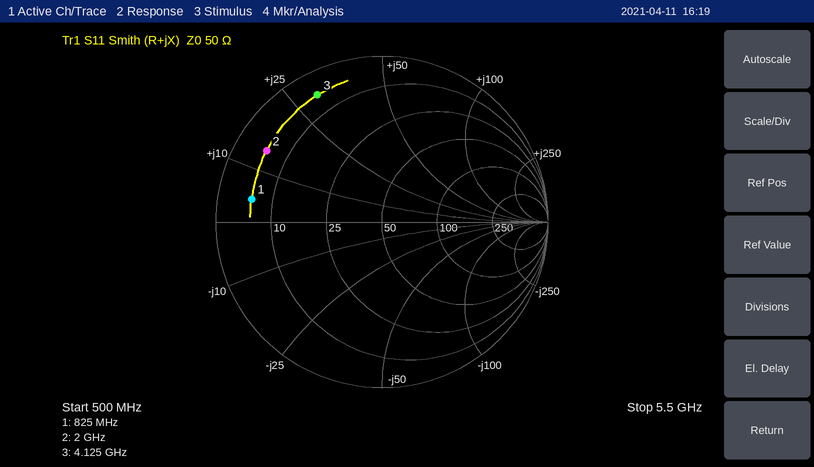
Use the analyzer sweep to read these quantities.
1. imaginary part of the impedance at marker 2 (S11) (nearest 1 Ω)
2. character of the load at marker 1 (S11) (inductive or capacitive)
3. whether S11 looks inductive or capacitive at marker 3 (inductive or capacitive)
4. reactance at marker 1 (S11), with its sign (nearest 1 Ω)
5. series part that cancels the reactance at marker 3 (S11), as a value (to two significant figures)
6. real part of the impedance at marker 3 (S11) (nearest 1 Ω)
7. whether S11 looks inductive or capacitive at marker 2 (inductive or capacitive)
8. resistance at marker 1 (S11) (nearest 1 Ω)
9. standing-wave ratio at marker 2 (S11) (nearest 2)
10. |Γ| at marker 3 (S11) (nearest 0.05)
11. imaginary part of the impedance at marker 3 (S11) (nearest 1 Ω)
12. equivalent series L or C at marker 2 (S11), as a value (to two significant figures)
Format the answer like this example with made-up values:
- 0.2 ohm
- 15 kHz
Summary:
- +14 Ω
- inductive
- inductive
- +4 Ω
- 1.3 pF
- 5 Ω
- inductive
- 6 Ω
- 10
- 0.85
- +30 Ω
- 1.1 nH
